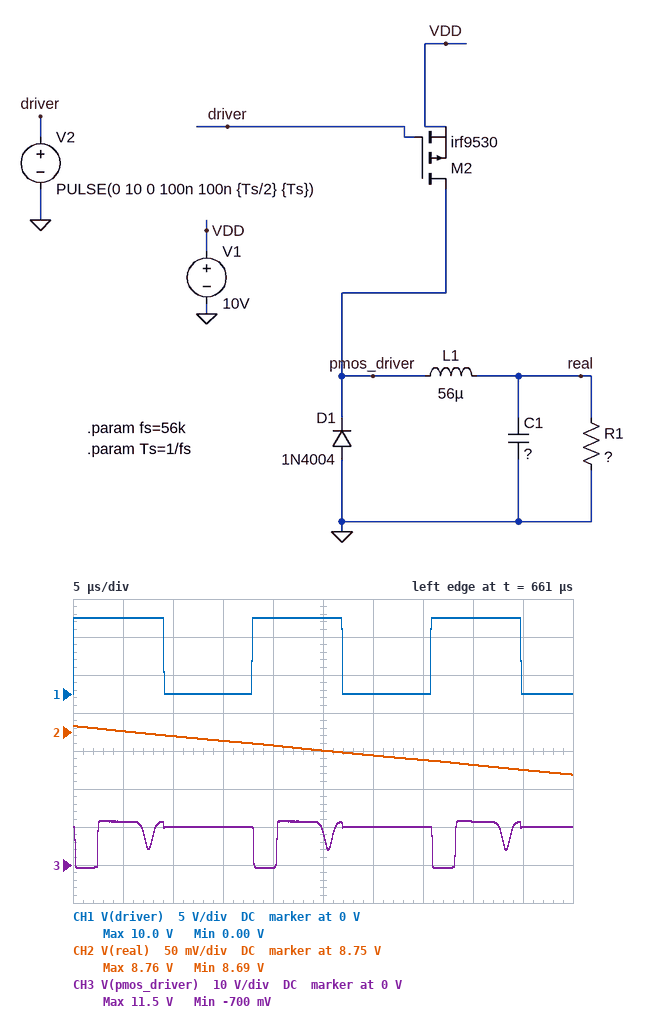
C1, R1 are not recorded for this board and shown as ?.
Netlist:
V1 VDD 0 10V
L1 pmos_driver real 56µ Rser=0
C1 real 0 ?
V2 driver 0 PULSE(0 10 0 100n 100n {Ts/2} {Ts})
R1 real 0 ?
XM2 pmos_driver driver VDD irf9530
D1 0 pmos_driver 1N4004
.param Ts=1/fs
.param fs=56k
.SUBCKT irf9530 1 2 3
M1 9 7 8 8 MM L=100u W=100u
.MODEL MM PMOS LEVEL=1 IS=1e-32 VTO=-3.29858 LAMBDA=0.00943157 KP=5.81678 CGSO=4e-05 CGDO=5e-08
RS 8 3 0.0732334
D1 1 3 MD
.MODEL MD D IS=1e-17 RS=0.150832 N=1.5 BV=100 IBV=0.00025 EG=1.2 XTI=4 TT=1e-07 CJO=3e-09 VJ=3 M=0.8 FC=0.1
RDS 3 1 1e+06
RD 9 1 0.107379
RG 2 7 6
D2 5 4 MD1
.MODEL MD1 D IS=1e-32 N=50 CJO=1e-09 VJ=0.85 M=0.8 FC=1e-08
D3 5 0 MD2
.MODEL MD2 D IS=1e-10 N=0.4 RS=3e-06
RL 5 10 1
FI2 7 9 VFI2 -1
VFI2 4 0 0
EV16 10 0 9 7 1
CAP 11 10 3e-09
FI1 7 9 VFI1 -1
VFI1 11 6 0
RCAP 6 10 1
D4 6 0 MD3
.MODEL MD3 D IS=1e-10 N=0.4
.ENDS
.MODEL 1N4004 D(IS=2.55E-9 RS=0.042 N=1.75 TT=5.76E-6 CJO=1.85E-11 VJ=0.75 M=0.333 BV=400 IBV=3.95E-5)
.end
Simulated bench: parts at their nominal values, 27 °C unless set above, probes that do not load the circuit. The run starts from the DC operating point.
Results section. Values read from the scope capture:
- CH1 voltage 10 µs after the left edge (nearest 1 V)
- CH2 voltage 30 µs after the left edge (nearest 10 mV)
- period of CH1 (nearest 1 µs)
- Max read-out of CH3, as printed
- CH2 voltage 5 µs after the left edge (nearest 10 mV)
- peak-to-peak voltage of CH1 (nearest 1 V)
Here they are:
0 V
8.72 V
18 µs
11.5 V
8.75 V
10 V
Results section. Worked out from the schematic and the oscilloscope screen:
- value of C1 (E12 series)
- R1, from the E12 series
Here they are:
1.2 mF
5.6 Ω
